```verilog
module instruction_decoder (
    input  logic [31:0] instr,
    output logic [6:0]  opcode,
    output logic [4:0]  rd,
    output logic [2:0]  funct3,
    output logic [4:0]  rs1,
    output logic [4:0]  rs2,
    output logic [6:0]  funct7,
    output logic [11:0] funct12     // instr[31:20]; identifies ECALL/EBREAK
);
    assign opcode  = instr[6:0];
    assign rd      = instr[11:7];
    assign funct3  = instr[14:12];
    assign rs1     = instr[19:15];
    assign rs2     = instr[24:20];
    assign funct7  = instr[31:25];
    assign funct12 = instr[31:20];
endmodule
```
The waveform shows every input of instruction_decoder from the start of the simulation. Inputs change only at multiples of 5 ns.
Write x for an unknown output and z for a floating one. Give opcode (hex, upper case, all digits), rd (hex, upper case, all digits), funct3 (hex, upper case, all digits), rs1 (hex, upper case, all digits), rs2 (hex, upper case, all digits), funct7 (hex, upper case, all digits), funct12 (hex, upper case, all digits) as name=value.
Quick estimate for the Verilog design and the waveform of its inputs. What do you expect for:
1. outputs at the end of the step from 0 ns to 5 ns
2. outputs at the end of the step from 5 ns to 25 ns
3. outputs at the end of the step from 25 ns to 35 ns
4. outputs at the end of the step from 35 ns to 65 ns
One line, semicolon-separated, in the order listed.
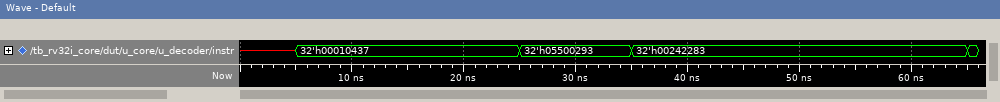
opcode=x, rd=x, funct3=x, rs1=x, rs2=x, funct7=x, funct12=x; opcode=37, rd=08, funct3=0, rs1=02, rs2=00, funct7=00, funct12=000; opcode=13, rd=05, funct3=0, rs1=00, rs2=15, funct7=02, funct12=055; opcode=03, rd=05, funct3=2, rs1=08, rs2=02, funct7=00, funct12=002
